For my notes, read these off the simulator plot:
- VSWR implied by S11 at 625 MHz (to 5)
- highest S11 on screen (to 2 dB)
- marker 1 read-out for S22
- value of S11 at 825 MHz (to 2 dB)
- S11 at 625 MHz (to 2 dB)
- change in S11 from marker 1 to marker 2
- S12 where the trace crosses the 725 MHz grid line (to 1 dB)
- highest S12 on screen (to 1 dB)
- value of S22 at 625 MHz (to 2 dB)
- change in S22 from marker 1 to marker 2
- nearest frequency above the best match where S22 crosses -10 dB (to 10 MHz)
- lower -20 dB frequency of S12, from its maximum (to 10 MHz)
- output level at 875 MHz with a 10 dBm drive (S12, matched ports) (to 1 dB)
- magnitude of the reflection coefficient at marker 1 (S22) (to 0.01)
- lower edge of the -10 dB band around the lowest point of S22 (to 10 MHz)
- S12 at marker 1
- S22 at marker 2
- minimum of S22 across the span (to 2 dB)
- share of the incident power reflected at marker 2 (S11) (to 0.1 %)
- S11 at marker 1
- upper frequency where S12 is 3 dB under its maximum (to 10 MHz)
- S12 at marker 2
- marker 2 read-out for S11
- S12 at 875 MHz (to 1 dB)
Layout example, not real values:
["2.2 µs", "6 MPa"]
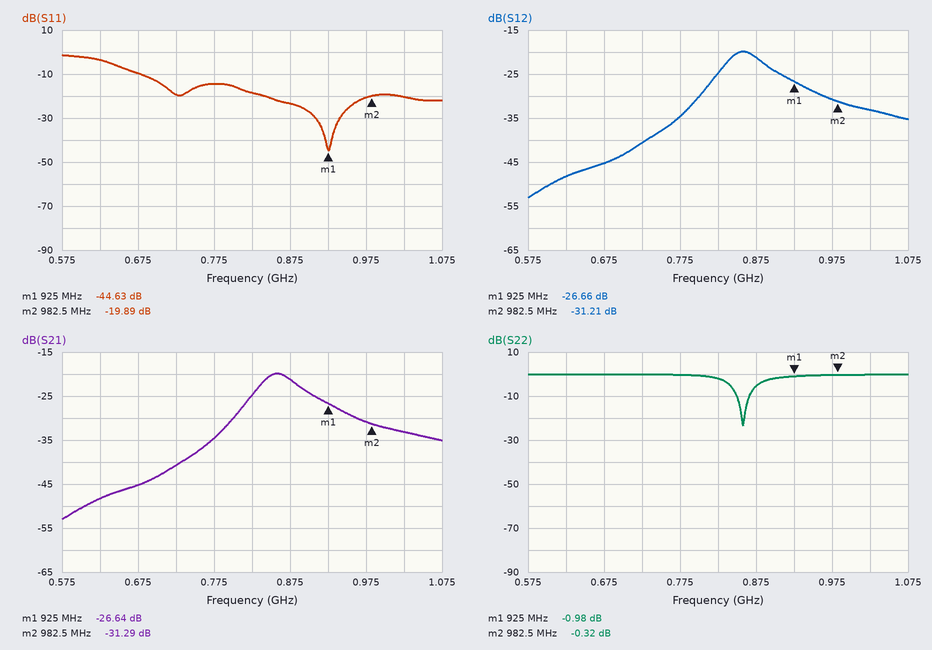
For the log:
["5", "-2 dB", "-0.98 dB", "-18 dB", "-4 dB", "24.74 dB", "-41 dB", "-20 dB", "0 dB", "0.66 dB", "870 MHz", "730 MHz", "-11 dBm", "0.89", "850 MHz", "-26.66 dB", "-0.32 dB", "-24 dB", "1.0 %", "-44.63 dB", "890 MHz", "-31.21 dB", "-19.89 dB", "-21 dB"]
